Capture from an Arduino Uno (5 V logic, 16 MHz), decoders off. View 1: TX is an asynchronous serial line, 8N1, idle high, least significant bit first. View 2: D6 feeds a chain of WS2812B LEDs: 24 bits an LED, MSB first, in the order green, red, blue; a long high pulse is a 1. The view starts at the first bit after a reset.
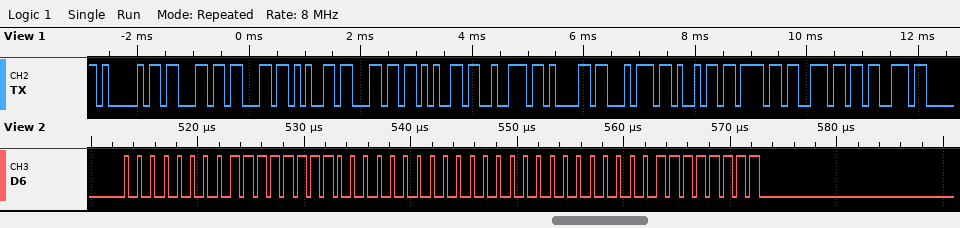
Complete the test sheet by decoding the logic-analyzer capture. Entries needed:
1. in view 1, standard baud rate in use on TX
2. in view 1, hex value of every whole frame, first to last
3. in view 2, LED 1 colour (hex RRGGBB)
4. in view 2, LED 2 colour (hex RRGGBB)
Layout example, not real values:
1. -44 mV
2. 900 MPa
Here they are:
1. 9600 baud
2. 41 63 63 65 6C 65 72 61 74 69 6F 6E 73
3. #FF0000
4. #0000FF
